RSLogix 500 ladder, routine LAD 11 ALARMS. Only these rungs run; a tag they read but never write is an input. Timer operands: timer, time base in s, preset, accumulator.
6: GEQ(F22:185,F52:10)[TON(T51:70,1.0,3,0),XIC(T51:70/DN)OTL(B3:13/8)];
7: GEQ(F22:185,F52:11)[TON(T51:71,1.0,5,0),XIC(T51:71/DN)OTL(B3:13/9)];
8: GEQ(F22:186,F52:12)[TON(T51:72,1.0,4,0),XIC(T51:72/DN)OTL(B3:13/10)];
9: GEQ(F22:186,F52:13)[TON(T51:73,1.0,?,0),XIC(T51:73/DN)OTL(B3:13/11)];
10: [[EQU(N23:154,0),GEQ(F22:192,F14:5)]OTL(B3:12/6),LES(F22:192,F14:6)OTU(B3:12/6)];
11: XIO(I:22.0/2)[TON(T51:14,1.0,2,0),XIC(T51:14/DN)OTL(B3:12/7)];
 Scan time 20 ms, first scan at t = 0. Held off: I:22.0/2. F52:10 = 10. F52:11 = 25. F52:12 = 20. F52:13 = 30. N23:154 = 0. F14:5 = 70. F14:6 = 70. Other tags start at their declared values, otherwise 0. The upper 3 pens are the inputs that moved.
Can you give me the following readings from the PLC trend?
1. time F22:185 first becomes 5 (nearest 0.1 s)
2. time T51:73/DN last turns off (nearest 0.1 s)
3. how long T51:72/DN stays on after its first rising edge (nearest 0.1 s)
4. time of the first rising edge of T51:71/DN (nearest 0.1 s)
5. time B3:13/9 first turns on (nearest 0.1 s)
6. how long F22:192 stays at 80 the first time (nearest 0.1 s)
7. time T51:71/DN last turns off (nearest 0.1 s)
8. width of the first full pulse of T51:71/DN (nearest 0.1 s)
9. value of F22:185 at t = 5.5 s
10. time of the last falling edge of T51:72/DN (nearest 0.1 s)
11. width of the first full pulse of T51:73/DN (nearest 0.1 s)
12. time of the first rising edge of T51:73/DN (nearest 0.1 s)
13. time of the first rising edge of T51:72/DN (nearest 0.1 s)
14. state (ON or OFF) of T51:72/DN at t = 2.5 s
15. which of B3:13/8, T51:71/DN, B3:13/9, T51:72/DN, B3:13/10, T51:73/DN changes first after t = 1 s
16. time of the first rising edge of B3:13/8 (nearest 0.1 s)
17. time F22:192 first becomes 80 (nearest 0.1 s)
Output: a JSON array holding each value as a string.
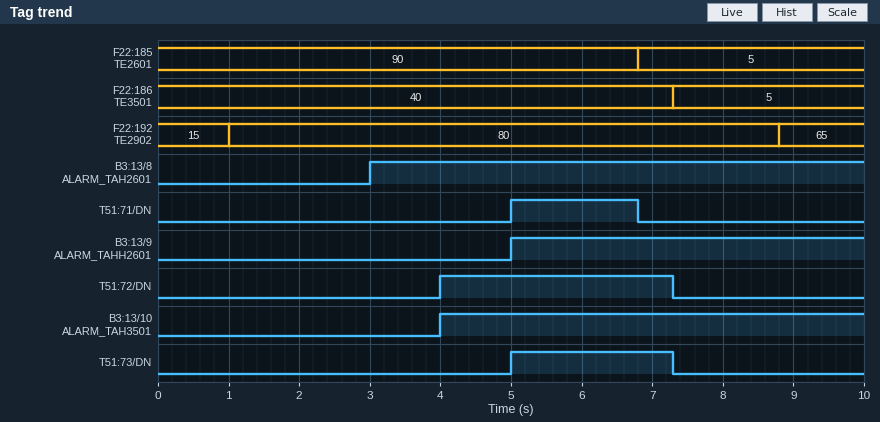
["6.8 s", "7.3 s", "3.3 s", "5.0 s", "5.0 s", "7.8 s", "6.8 s", "1.8 s", "90", "7.3 s", "2.3 s", "5.0 s", "4.0 s", "OFF", "B3:13/8", "3.0 s", "1.0 s"]
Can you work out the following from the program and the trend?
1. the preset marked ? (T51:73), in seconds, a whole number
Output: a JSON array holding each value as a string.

["5 s"]
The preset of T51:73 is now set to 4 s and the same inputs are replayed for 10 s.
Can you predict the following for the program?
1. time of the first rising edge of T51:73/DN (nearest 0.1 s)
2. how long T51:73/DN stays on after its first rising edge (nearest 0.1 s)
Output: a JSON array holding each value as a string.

["4.0 s", "3.3 s"]
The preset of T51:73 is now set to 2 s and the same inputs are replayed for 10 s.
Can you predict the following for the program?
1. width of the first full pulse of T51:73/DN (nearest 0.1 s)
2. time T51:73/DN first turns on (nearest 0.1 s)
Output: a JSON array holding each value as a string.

["5.3 s", "2.0 s"]
